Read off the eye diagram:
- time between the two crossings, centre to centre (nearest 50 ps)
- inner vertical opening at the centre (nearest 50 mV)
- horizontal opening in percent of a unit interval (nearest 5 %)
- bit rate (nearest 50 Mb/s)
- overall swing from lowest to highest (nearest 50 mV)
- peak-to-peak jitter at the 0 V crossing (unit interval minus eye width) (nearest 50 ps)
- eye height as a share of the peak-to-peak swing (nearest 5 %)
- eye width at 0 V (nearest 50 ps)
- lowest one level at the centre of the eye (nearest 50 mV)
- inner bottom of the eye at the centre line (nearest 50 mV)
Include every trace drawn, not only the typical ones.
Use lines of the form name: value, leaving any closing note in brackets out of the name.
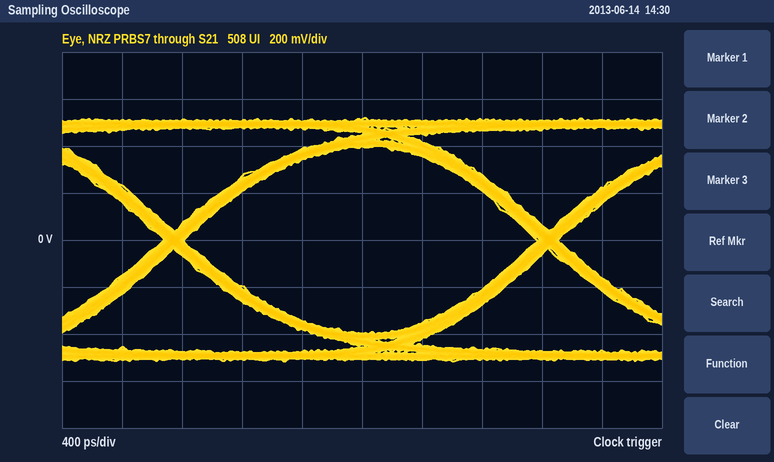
time between the two crossings, centre to centre: 2.50 ns
inner vertical opening at the centre: 800 mV
horizontal opening in percent of a unit interval: 95 %
bit rate: 400 Mb/s
overall swing from lowest to highest: 1.05 V
peak-to-peak jitter at the 0 V crossing (unit interval minus eye width): 150 ps
eye height as a share of the peak-to-peak swing: 75 %
eye width at 0 V: 2.35 ns
lowest one level at the centre of the eye: 400 mV
inner bottom of the eye at the centre line: -400 mV
